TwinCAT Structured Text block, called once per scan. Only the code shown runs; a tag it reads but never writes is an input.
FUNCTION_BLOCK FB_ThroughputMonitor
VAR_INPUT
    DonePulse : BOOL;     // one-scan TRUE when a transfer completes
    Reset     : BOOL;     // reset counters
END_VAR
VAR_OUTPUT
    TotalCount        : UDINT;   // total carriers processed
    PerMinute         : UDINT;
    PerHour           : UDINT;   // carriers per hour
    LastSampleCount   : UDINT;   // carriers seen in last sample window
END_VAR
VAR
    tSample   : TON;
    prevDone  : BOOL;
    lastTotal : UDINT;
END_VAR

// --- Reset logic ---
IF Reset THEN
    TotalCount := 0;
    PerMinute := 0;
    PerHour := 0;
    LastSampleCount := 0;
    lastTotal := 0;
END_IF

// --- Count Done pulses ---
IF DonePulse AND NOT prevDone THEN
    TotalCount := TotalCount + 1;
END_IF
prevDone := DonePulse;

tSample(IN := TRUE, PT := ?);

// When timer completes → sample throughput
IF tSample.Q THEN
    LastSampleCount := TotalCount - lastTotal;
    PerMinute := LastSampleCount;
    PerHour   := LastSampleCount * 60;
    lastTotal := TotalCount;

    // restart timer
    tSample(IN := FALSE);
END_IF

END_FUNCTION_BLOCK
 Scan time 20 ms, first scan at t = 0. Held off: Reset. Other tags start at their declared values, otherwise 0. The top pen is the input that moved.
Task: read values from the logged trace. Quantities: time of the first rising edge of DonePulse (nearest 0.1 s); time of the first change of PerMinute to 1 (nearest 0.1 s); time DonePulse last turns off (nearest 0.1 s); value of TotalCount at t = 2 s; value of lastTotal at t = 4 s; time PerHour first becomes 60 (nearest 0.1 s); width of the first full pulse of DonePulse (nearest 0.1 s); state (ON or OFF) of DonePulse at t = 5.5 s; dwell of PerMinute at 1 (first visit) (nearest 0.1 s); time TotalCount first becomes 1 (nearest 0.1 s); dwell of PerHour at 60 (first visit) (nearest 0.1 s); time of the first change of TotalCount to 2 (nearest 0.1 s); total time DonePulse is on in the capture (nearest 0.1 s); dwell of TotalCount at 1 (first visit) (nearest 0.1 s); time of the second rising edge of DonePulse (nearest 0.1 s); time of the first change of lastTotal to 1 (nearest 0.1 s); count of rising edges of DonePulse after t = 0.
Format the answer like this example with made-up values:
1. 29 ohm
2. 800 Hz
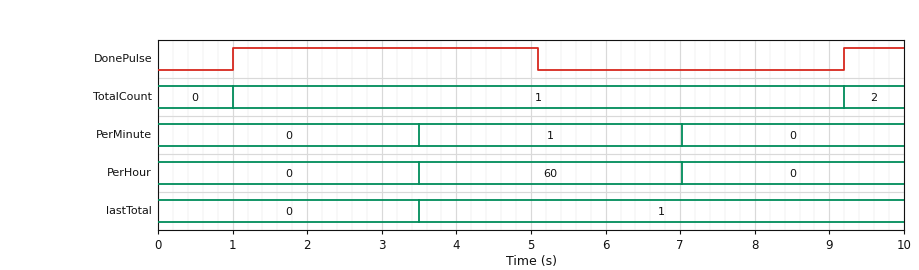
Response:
1. 1.0 s
2. 3.5 s
3. 5.1 s
4. 1
5. 1
6. 3.5 s
7. 4.1 s
8. OFF
9. 3.5 s
10. 1.0 s
11. 3.5 s
12. 9.2 s
13. 4.9 s
14. 8.2 s
15. 9.2 s
16. 3.5 s
17. 2
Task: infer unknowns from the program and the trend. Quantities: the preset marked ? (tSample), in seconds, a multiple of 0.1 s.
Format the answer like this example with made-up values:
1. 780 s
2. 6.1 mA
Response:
1. 3.5 s
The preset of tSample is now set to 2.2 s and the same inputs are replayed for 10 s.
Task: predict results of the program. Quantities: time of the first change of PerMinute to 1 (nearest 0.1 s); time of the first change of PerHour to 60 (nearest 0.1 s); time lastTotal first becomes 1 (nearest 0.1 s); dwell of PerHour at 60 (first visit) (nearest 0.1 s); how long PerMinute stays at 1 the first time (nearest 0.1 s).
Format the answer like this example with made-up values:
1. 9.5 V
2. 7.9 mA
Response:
1. 2.2 s
2. 2.2 s
3. 2.2 s
4. 2.2 s
5. 2.2 s
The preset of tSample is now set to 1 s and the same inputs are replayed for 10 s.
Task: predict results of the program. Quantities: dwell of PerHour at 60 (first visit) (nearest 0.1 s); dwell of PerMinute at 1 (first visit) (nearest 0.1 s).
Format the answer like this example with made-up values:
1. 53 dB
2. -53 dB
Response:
1. 1.0 s
2. 1.0 s
